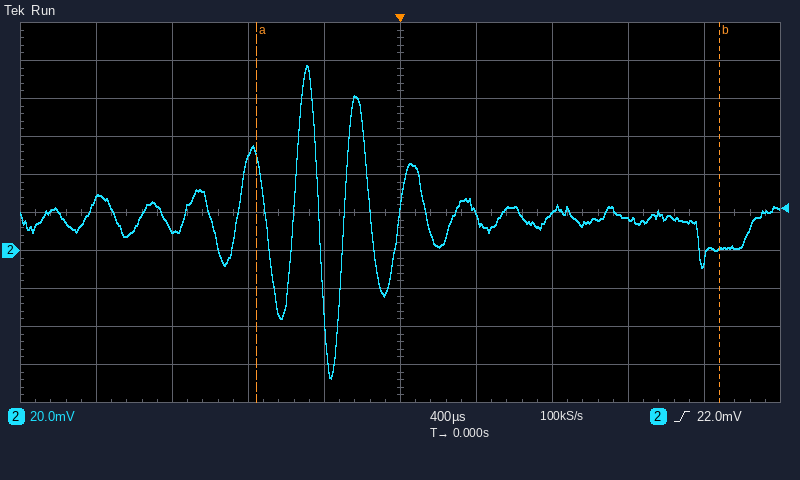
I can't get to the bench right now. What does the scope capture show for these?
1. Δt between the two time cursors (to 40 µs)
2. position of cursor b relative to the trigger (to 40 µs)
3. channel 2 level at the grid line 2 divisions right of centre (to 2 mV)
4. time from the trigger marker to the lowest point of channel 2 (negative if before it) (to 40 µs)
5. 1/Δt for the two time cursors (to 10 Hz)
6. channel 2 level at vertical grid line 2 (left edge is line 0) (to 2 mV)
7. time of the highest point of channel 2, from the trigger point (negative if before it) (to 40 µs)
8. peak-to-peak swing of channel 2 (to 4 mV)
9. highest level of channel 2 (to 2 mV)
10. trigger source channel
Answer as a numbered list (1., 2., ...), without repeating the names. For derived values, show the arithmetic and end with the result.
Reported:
1. 2.44 ms
2. +1.68 ms
3. 20 mV
4. -360 µs
5. 1 / 2.44 ms ≈ 410 Hz
6. 12 mV
7. -480 µs
8. 164 mV
9. 98 mV
10. channel 2
